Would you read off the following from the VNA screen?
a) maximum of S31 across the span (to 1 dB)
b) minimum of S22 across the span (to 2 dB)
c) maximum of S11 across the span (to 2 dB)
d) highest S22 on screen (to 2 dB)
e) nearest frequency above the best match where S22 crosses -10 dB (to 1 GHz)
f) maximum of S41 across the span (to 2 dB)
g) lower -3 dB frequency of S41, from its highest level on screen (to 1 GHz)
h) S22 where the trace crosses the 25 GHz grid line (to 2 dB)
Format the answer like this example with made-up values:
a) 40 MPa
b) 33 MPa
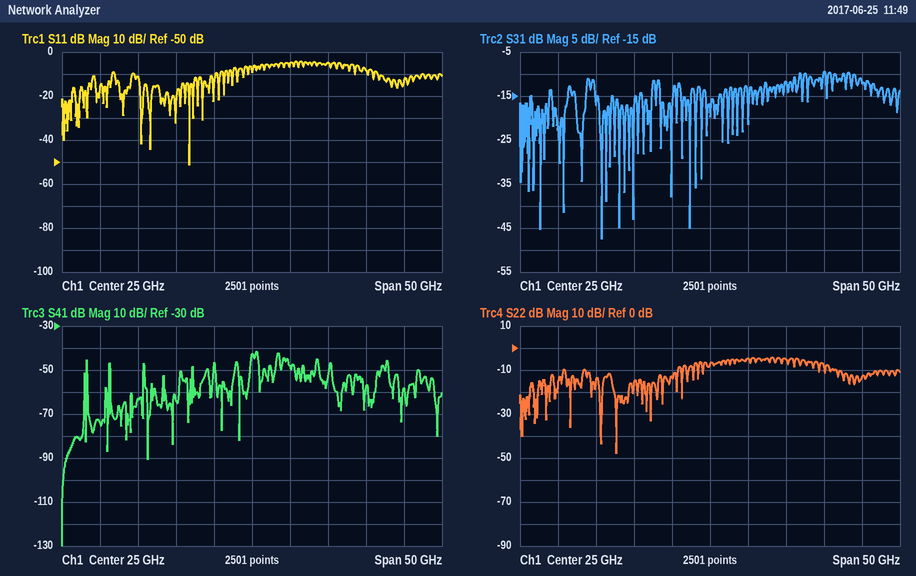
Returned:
a) -9 dB
b) -48 dB
c) -4 dB
d) -4 dB
e) 21 GHz
f) -42 dB
g) 25 GHz
h) -8 dB
